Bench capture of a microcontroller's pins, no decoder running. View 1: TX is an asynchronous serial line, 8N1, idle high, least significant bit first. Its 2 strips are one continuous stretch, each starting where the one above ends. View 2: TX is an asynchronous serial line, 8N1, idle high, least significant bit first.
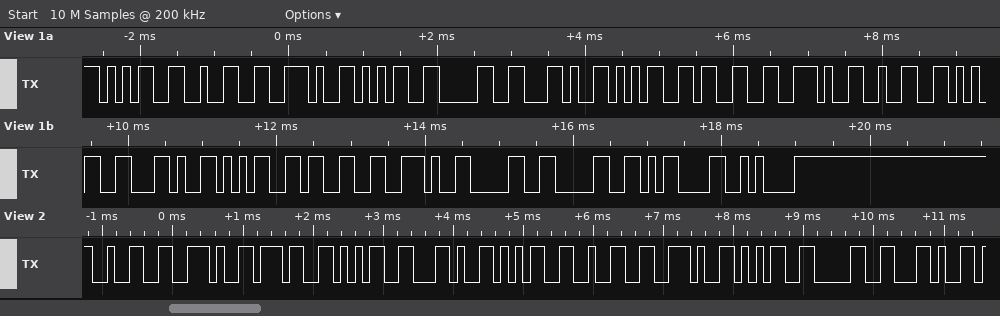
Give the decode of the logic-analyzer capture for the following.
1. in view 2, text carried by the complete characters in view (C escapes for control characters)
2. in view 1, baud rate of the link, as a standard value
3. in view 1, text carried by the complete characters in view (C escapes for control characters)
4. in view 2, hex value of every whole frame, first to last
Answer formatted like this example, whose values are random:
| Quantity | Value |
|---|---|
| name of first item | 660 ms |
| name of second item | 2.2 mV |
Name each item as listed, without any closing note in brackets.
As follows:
| Quantity | Value |
|---|---|
| in view 2, text carried by the complete characters in view | "2.75,52.50," |
| in view 1, baud rate of the link, as a standard value | 9600 baud |
| in view 1, text carried by the complete characters in view | "52.50,53.25,53.00\r\n" |
| in view 2, hex value of every whole frame, first to last | 32 2E 37 35 2C 35 32 2E 35 30 2C |
